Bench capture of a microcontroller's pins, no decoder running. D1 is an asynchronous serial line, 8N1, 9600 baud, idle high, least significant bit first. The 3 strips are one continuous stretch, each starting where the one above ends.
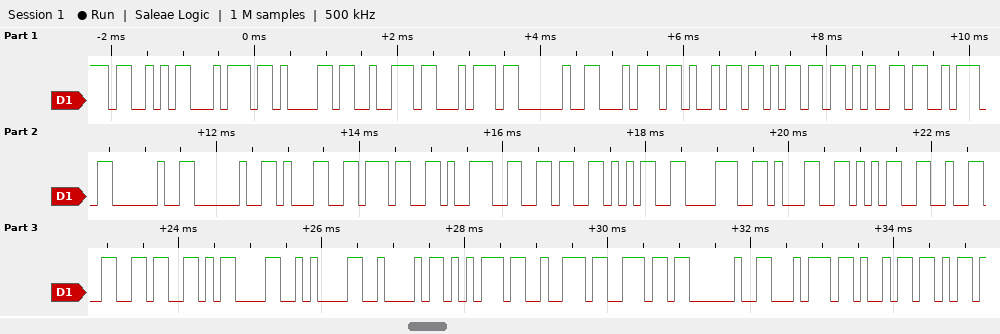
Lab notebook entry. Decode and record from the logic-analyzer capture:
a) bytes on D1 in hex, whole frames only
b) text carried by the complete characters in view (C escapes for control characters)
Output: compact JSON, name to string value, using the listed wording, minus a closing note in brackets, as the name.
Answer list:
{"bytes on D1 in hex, whole frames only": "53 74 61 72 74 20 74 69 6D 65 3A 20 20 31 37 39 36 35 38 31 35 32 36 0D 0A 42 75 72 6E 20 74 69", "text carried by the complete characters in view": "\"Start time:  1796581526\\r\\nBurn ti\""}
